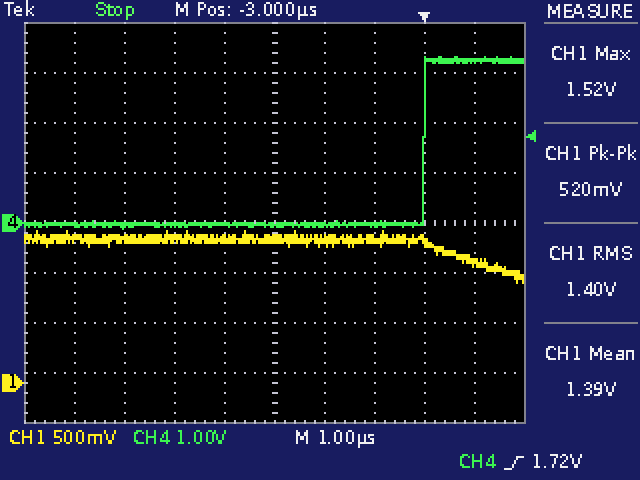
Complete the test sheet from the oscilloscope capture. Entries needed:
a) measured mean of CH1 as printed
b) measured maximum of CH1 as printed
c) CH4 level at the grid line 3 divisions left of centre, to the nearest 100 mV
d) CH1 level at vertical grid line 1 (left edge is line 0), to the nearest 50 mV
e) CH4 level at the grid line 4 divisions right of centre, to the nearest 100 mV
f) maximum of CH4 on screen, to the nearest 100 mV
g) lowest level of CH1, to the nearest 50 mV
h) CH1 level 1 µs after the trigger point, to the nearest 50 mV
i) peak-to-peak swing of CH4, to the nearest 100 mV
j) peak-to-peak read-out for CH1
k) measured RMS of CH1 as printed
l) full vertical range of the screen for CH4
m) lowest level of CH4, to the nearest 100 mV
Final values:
1.39 V
1.52 V
-100 mV
1.45 V
3.2 V
3.3 V
1.00 V
1.20 V
3.4 V
520 mV
1.40 V
8 V
-100 mV
